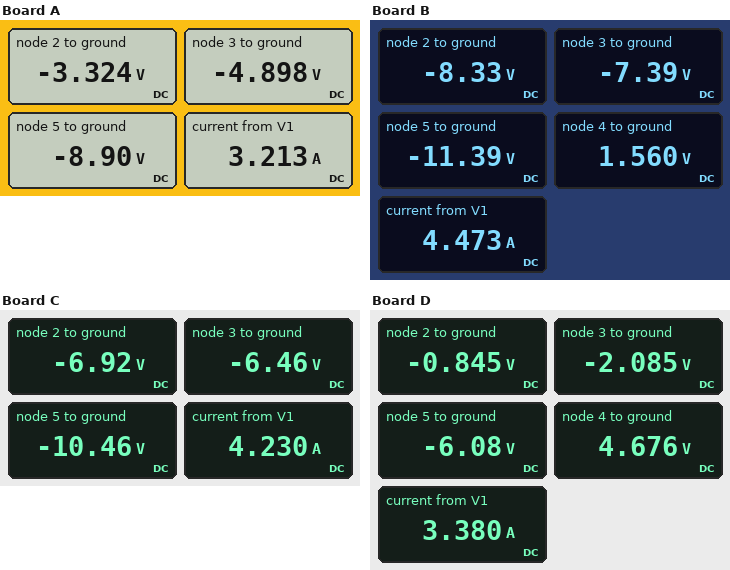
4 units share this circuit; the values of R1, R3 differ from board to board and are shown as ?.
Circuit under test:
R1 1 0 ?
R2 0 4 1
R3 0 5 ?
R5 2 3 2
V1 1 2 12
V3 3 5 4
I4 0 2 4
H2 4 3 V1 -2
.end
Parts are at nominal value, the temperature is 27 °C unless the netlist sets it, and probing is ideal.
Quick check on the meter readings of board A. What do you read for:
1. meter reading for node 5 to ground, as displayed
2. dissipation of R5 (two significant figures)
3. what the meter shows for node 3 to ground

-8.90 V
1.2 W
-4.898 V
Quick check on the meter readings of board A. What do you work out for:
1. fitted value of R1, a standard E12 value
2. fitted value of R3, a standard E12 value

2.7 Ω
12 Ω
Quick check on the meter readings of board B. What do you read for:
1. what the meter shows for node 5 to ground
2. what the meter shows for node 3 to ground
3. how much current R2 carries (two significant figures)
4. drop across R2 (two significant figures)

-11.39 V
-7.39 V
1.6 A
1.6 V
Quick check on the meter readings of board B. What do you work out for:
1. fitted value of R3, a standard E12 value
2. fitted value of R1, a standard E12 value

5.6 Ω
0.82 Ω
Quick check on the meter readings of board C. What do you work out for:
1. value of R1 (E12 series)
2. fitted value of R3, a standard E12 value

1.2 Ω
4.7 Ω
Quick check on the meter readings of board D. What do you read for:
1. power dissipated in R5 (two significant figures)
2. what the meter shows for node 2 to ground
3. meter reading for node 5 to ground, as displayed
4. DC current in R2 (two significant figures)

770 mW
-0.845 V
-6.08 V
4.7 A
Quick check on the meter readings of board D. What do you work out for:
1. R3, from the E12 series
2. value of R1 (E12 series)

1.5 Ω
3.3 Ω
